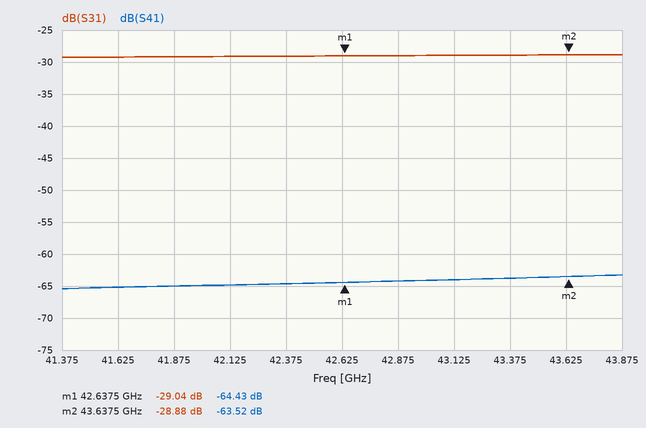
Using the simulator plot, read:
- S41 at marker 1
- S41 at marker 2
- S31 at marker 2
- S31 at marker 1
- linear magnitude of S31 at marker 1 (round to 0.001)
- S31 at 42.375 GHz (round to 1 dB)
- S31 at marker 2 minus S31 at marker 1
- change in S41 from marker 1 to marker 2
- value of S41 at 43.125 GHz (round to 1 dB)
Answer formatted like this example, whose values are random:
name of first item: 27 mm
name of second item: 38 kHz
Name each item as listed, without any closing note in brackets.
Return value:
S41 at marker 1: -64.43 dB
S41 at marker 2: -63.52 dB
S31 at marker 2: -28.88 dB
S31 at marker 1: -29.04 dB
linear magnitude of S31 at marker 1: 0.035
S31 at 42.375 GHz: -29 dB
S31 at marker 2 minus S31 at marker 1: 0.16 dB
change in S41 from marker 1 to marker 2: 0.91 dB
value of S41 at 43.125 GHz: -64 dB
